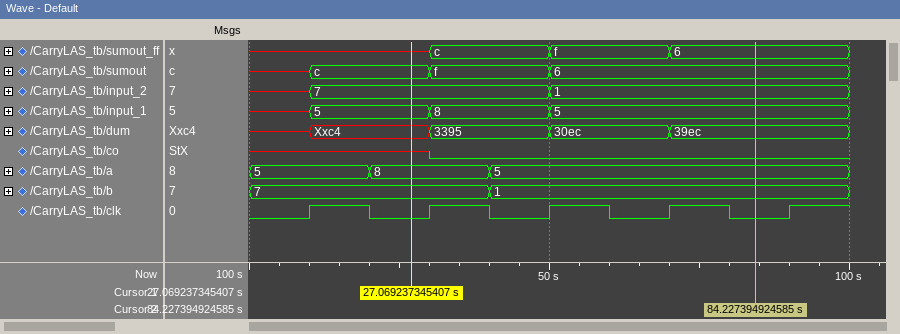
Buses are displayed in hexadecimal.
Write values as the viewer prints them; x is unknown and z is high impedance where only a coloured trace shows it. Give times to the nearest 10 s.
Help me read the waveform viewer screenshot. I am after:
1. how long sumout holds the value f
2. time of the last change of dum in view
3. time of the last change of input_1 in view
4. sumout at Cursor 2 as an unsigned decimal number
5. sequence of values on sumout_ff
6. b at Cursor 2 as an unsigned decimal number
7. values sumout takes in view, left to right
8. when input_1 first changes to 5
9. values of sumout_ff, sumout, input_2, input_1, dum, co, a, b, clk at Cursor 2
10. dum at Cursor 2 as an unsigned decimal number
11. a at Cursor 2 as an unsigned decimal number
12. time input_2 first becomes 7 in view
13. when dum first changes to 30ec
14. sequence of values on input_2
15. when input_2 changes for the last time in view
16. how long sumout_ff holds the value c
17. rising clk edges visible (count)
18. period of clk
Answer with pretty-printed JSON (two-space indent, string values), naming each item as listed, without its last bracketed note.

{
  "how long sumout holds the value f": "20 s",
  "time of the last change of dum in view": "70 s",
  "time of the last change of input_1 in view": "50 s",
  "sumout at Cursor 2 as an unsigned decimal number": "6",
  "sequence of values on sumout_ff": "x, c, f, 6",
  "b at Cursor 2 as an unsigned decimal number": "1",
  "values sumout takes in view, left to right": "x, c, f, 6",
  "when input_1 first changes to 5": "10 s",
  "values of sumout_ff, sumout, input_2, input_1, dum, co, a, b, clk at Cursor 2": "sumout_ff=6, sumout=6, input_2=1, input_1=5, dum=39ec, co=0, a=5, b=1, clk=0",
  "dum at Cursor 2 as an unsigned decimal number": "14828",
  "a at Cursor 2 as an unsigned decimal number": "5",
  "time input_2 first becomes 7 in view": "10 s",
  "when dum first changes to 30ec": "50 s",
  "sequence of values on input_2": "x, 7, 1",
  "when input_2 changes for the last time in view": "50 s",
  "how long sumout_ff holds the value c": "20 s",
  "rising clk edges visible": "5",
  "period of clk": "20 s"
}
